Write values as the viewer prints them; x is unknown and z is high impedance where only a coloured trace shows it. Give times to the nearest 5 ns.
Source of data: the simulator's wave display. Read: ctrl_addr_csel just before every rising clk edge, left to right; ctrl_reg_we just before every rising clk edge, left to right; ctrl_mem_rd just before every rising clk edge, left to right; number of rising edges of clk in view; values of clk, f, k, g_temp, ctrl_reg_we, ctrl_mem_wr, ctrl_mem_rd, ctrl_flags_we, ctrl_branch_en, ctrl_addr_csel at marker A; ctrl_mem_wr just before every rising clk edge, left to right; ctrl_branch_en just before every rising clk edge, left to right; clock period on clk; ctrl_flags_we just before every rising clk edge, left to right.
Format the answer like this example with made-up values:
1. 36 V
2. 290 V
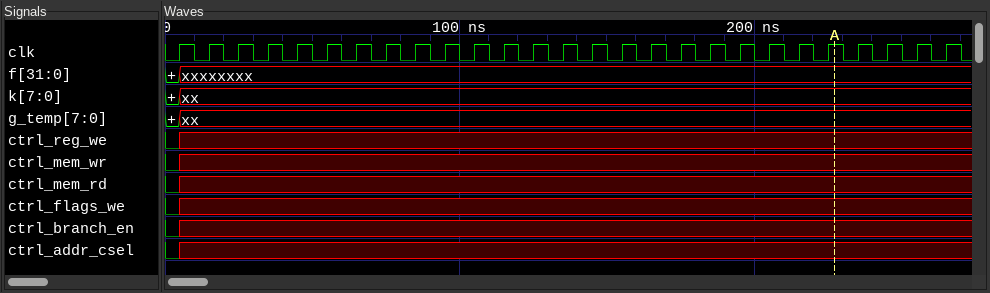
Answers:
1. 0 x x x x x x x x x x x x x x x x x x x x x x x x x x
2. 0 x x x x x x x x x x x x x x x x x x x x x x x x x x
3. 0 x x x x x x x x x x x x x x x x x x x x x x x x x x
4. 27
5. clk=1, f=xxxxxxxx, k=xx, g_temp=xx, ctrl_reg_we=x, ctrl_mem_wr=x, ctrl_mem_rd=x, ctrl_flags_we=x, ctrl_branch_en=x, ctrl_addr_csel=x
6. 0 x x x x x x x x x x x x x x x x x x x x x x x x x x
7. 0 x x x x x x x x x x x x x x x x x x x x x x x x x x
8. 10 ns
9. 0 x x x x x x x x x x x x x x x x x x x x x x x x x x
